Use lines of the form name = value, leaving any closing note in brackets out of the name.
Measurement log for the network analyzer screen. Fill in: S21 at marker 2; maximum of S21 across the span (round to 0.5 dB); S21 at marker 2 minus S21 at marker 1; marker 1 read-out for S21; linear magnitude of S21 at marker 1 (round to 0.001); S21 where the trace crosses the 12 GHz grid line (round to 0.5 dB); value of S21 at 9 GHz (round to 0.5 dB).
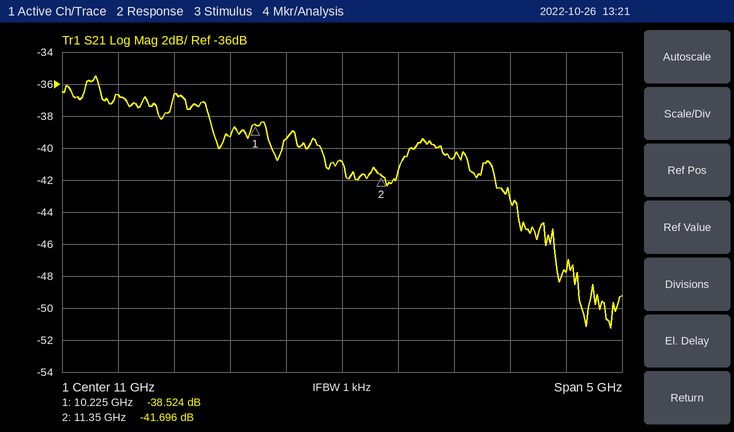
S21 at marker 2 = -41.696 dB
maximum of S21 across the span = -35.5 dB
S21 at marker 2 minus S21 at marker 1 = -3.172 dB
marker 1 read-out for S21 = -38.524 dB
linear magnitude of S21 at marker 1 = 0.012
S21 where the trace crosses the 12 GHz grid line = -40.5 dB
value of S21 at 9 GHz = -36.5 dB
